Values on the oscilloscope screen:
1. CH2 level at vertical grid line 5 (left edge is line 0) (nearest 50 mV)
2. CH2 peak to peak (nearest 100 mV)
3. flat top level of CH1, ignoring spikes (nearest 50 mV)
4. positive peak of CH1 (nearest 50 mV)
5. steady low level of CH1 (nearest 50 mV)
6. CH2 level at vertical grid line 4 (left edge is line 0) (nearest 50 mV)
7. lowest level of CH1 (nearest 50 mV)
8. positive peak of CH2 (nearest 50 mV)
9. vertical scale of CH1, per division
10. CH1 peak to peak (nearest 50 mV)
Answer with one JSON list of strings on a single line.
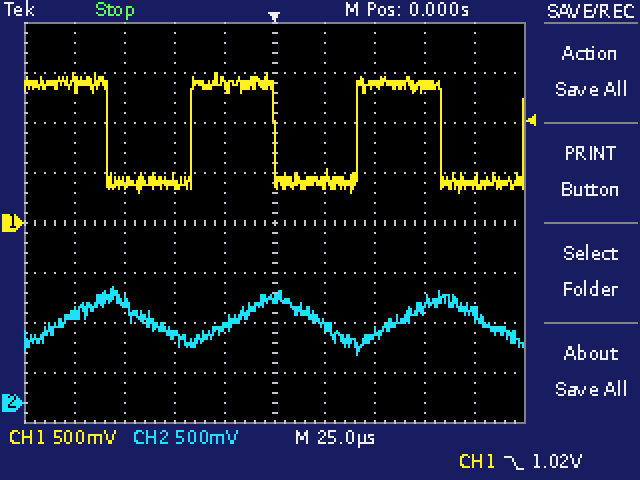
["1.05 V", "700 mV", "1.40 V", "1.50 V", "400 mV", "750 mV", "300 mV", "1.15 V", "500 mV", "1.20 V"]
